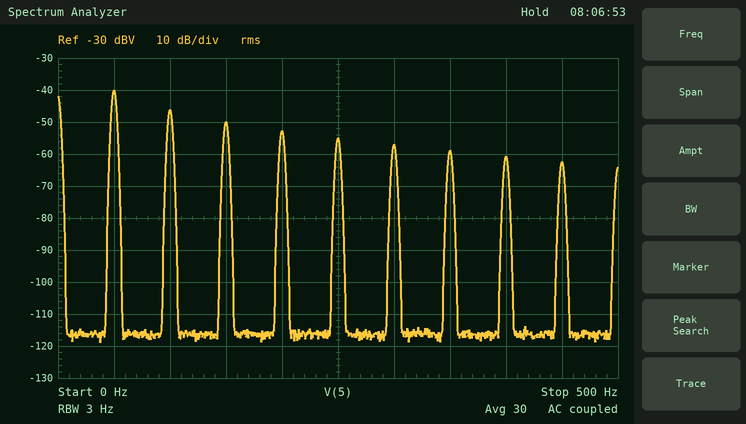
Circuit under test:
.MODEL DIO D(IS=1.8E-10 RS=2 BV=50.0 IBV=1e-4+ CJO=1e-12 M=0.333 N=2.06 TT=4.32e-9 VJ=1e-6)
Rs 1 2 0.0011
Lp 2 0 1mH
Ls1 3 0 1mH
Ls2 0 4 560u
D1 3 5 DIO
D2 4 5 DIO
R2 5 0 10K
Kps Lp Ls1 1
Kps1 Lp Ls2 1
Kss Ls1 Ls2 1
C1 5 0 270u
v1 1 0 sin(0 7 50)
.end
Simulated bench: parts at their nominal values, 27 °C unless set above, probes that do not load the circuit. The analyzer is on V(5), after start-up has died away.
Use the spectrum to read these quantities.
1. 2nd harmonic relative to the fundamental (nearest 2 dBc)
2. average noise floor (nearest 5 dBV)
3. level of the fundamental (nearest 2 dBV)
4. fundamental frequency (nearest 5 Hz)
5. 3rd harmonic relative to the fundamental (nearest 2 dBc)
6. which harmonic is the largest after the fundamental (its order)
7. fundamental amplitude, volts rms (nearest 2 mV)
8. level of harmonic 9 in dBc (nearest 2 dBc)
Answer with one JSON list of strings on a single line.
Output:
["-6 dBc", "-115 dBV", "-40 dBV", "50 Hz", "-10 dBc", "2", "10 mV", "-22 dBc"]
